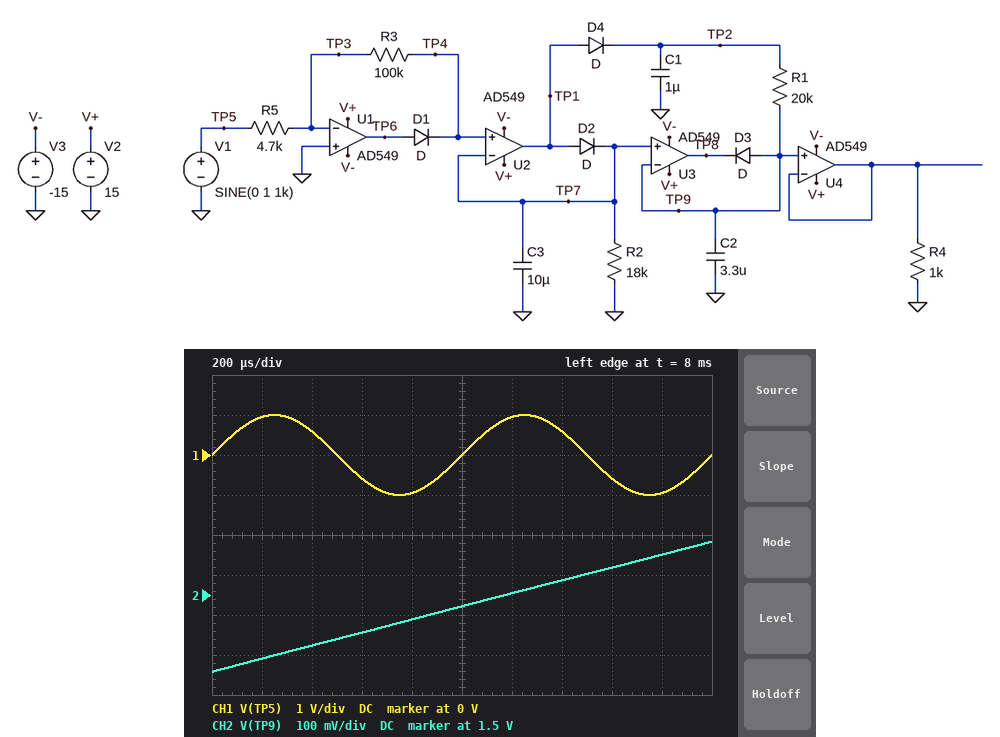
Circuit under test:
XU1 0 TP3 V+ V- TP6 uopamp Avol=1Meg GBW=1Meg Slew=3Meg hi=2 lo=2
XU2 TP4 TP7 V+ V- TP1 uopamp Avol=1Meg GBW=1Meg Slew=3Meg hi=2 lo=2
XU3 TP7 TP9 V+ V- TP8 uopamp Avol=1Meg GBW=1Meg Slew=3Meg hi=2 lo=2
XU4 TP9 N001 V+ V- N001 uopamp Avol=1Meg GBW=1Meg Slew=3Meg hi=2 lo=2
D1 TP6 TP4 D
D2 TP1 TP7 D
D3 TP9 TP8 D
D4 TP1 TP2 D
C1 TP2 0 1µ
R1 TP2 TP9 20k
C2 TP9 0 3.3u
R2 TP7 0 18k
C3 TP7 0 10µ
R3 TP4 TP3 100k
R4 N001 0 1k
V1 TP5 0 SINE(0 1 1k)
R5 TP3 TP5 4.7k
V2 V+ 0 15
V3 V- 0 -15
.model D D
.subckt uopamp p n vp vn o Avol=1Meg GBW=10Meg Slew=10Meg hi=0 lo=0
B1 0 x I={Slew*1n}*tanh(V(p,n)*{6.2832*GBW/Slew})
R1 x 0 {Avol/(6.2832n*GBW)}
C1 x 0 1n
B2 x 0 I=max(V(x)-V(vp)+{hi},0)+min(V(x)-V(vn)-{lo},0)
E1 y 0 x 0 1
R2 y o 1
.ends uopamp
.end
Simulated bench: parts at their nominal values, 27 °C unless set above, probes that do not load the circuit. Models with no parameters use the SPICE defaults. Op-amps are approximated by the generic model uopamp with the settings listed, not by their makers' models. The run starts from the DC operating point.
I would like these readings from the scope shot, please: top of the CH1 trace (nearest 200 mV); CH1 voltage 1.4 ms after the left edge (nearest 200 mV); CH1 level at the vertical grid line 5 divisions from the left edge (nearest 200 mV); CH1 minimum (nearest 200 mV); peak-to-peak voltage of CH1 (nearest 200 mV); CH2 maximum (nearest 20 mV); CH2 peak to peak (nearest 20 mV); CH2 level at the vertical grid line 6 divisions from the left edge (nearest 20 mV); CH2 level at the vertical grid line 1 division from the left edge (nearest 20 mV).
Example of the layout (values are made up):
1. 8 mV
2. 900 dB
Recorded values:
1. 1.0 V
2. 600 mV
3. 0 V
4. -1.0 V
5. 2.0 V
6. 1.64 V
7. 320 mV
8. 1.50 V
9. 1.34 V
